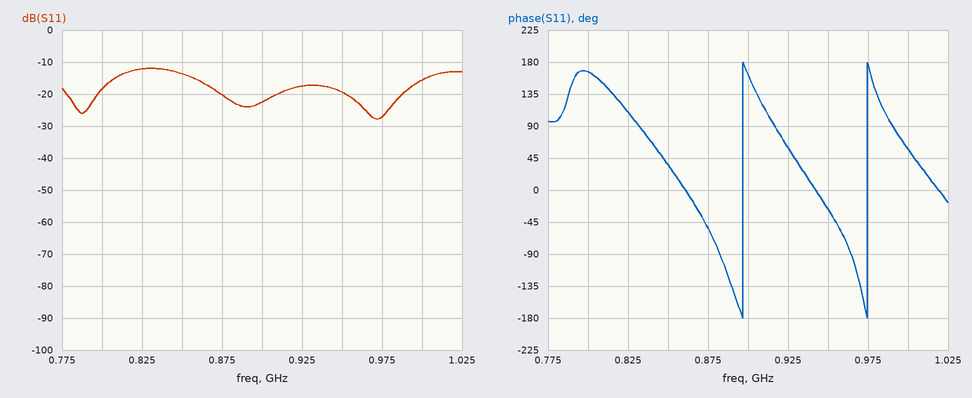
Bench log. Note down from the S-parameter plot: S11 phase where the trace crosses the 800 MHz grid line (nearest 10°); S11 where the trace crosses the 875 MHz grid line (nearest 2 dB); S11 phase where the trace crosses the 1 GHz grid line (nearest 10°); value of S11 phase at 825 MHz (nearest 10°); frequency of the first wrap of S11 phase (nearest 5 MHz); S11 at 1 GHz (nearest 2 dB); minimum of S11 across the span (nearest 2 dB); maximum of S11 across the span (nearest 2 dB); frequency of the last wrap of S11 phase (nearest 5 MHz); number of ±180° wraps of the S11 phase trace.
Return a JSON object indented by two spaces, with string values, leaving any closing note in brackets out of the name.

{
  "S11 phase where the trace crosses the 800 MHz grid line": "170°",
  "S11 where the trace crosses the 875 MHz grid line": "-20 dB",
  "S11 phase where the trace crosses the 1 GHz grid line": "60°",
  "value of S11 phase at 825 MHz": "110°",
  "frequency of the first wrap of S11 phase": "895 MHz",
  "S11 at 1 GHz": "-16 dB",
  "minimum of S11 across the span": "-28 dB",
  "maximum of S11 across the span": "-12 dB",
  "frequency of the last wrap of S11 phase": "975 MHz",
  "number of ±180° wraps of the S11 phase trace": "2"
}
